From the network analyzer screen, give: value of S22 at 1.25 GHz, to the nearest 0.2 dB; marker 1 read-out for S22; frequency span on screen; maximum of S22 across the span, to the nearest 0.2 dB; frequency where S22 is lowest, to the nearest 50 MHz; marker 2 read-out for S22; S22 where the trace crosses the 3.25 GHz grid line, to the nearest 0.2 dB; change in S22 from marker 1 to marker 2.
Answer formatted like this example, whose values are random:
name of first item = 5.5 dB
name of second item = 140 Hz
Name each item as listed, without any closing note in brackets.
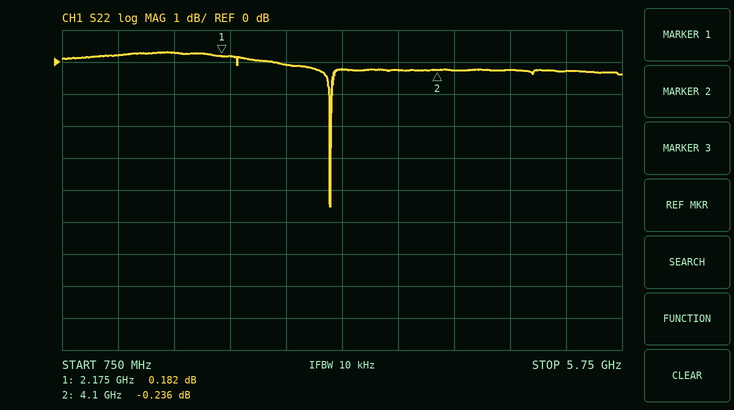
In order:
value of S22 at 1.25 GHz, to the nearest 0.2 dB = 0.2 dB
marker 1 read-out for S22 = 0.182 dB
frequency span on screen = 5 GHz
maximum of S22 across the span, to the nearest 0.2 dB = 0.4 dB
frequency where S22 is lowest, to the nearest 50 MHz = 3.15 GHz
marker 2 read-out for S22 = -0.236 dB
S22 where the trace crosses the 3.25 GHz grid line, to the nearest 0.2 dB = -0.2 dB
change in S22 from marker 1 to marker 2 = -0.418 dB
